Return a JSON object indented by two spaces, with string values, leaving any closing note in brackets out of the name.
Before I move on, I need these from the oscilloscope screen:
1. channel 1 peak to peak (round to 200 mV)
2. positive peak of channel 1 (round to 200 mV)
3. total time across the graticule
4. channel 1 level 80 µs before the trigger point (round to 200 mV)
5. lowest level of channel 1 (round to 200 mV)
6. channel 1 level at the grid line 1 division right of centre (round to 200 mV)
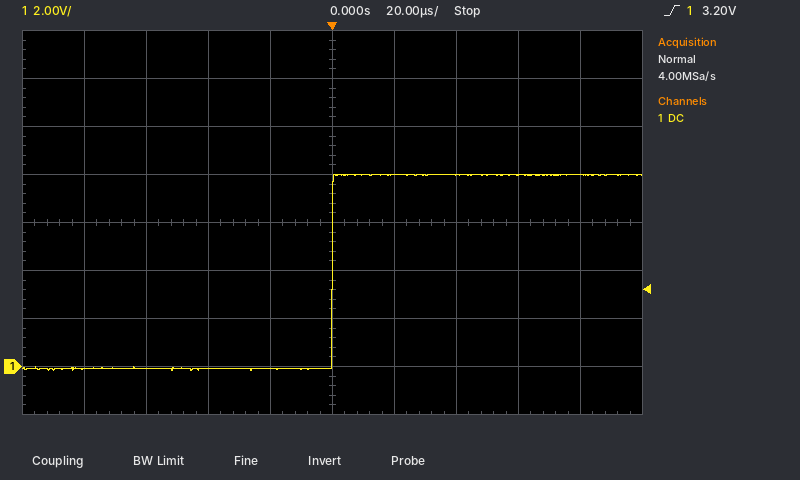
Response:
{
  "channel 1 peak to peak": "8.2 V",
  "positive peak of channel 1": "8.0 V",
  "total time across the graticule": "200 µs",
  "channel 1 level 80 µs before the trigger point": "-200 mV",
  "lowest level of channel 1": "-200 mV",
  "channel 1 level at the grid line 1 division right of centre": "8.0 V"
}
